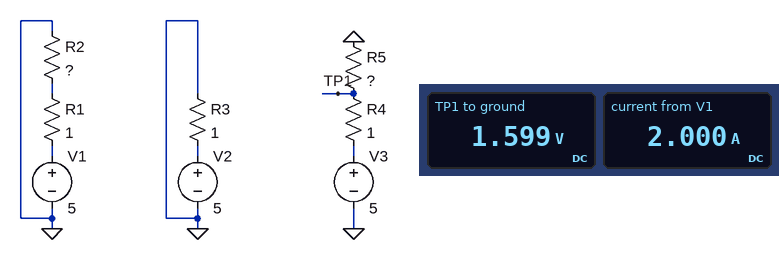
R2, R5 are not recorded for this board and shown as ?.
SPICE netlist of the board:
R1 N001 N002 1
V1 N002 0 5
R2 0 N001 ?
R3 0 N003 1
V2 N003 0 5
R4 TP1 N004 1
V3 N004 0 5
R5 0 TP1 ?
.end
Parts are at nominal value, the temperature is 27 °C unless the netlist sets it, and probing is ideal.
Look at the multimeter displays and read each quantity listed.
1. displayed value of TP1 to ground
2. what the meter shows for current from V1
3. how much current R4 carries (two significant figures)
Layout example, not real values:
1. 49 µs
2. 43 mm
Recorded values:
1. 1.599 V
2. 2.000 A
3. 3.4 A
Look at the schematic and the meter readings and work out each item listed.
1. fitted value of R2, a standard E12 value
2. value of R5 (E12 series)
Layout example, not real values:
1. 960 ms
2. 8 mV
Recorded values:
1. 1.5 Ω
2. 0.47 Ω
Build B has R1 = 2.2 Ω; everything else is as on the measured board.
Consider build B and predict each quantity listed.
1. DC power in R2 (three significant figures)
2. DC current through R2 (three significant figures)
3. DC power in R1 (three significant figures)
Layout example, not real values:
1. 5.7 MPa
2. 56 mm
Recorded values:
1. 2.74 W
2. 1.35 A
3. 4.02 W
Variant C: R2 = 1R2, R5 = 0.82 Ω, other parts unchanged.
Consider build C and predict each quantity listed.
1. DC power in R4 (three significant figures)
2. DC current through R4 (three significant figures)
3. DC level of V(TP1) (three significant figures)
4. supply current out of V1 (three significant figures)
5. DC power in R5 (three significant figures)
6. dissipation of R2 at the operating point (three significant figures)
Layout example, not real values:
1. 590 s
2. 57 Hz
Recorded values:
1. 7.55 W
2. 2.75 A
3. 2.25 V
4. 2.27 A
5. 6.19 W
6. 6.20 W
